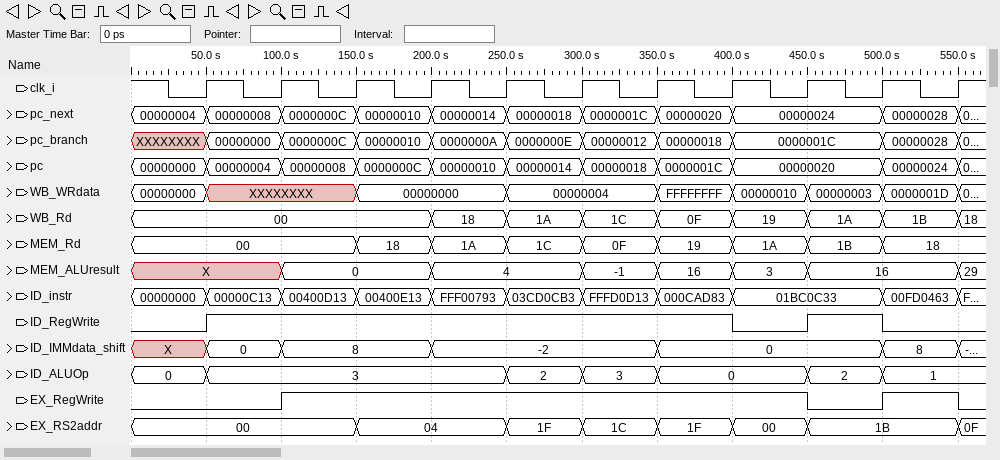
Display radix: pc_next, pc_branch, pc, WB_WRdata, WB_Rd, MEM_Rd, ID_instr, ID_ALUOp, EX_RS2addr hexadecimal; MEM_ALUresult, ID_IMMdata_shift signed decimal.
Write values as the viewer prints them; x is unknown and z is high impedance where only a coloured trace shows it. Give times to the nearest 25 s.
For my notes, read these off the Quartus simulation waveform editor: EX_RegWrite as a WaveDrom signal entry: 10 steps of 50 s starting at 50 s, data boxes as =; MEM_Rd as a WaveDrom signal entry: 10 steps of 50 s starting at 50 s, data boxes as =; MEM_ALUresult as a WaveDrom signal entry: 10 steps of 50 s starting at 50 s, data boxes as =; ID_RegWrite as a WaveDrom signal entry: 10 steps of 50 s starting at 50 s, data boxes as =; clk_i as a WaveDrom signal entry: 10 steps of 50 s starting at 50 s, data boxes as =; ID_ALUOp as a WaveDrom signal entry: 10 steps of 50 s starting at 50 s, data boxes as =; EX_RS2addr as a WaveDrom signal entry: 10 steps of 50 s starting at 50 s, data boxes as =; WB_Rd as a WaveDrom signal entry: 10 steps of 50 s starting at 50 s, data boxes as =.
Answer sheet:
{name: 'EX_RegWrite', wave: '01......01'}
{name: 'MEM_Rd', wave: '=.========', data: '00 18 1A 1C 0F 19 1A 1B 18'}
{name: 'MEM_ALUresult', wave: 'x=.=.====.', data: '0 4 -1 16 3 16'}
{name: 'ID_RegWrite', wave: '1......010'}
{name: 'clk_i', wave: 'p.........'}
{name: 'ID_ALUOp', wave: '=...===.==', data: '3 2 3 0 2 1'}
{name: 'EX_RS2addr', wave: '=.=.=====.', data: '00 04 1F 1C 1F 00 1B'}
{name: 'WB_Rd', wave: '=..=======', data: '00 18 1A 1C 0F 19 1A 1B'}
